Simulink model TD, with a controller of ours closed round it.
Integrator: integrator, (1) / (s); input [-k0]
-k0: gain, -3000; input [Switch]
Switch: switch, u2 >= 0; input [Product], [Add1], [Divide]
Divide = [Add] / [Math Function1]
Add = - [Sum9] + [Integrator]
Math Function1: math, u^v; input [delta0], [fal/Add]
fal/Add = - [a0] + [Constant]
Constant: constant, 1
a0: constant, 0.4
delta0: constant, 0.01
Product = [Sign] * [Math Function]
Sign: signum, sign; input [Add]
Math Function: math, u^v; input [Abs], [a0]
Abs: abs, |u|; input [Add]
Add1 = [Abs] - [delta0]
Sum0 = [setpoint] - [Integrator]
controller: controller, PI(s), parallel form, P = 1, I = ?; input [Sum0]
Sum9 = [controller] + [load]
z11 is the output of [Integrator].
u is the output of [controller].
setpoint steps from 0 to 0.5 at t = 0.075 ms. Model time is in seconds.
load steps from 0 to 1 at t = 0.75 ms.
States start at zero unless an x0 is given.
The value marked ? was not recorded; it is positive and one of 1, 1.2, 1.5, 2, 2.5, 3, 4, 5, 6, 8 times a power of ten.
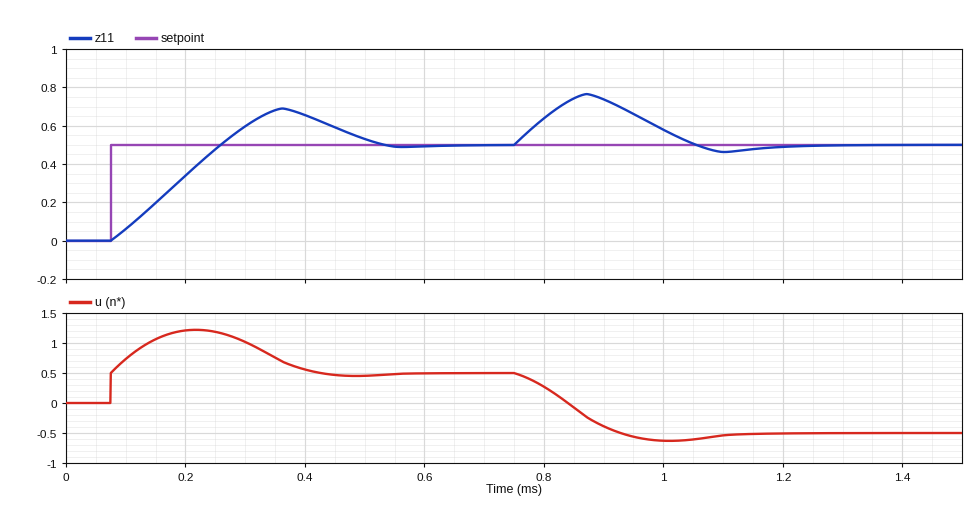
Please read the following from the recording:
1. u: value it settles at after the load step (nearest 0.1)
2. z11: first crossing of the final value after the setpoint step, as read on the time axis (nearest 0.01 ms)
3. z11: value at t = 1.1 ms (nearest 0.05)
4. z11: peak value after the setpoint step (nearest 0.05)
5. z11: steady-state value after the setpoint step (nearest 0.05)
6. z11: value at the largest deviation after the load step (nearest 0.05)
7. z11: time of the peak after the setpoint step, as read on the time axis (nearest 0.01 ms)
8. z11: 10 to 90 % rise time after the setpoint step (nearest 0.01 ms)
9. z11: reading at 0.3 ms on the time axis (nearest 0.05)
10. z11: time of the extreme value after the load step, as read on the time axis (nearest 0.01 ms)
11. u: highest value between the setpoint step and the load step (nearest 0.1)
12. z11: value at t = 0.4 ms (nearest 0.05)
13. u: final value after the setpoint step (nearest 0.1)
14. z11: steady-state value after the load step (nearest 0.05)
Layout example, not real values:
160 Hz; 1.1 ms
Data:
-0.5; 0.26 ms; 0.45; 0.70; 0.50; 0.75; 0.36 ms; 0.14 ms; 0.60; 0.87 ms; 1.2; 0.65; 0.5; 0.50
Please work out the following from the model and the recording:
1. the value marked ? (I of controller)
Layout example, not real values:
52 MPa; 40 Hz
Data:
25000
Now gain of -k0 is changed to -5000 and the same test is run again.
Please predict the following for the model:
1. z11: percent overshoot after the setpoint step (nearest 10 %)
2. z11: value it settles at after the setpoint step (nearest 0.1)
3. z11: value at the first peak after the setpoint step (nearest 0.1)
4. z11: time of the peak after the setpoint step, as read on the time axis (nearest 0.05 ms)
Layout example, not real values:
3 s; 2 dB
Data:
20 %; 0.5; 0.6; 0.25 ms
